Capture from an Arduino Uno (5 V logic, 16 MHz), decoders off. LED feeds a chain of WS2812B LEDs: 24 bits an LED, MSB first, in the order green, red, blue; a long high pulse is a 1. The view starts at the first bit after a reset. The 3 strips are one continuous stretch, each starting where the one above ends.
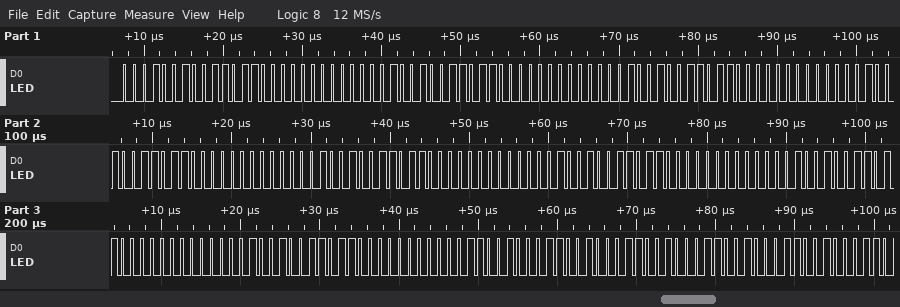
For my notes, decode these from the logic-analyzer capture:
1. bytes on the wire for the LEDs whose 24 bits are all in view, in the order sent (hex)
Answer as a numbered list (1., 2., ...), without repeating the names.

1. 12 6C 00 12 6C 00 12 6C 00 12 6C 00 12 6C 00 12 6C 00 12 6C 00 12 6C 00 64 64 64
